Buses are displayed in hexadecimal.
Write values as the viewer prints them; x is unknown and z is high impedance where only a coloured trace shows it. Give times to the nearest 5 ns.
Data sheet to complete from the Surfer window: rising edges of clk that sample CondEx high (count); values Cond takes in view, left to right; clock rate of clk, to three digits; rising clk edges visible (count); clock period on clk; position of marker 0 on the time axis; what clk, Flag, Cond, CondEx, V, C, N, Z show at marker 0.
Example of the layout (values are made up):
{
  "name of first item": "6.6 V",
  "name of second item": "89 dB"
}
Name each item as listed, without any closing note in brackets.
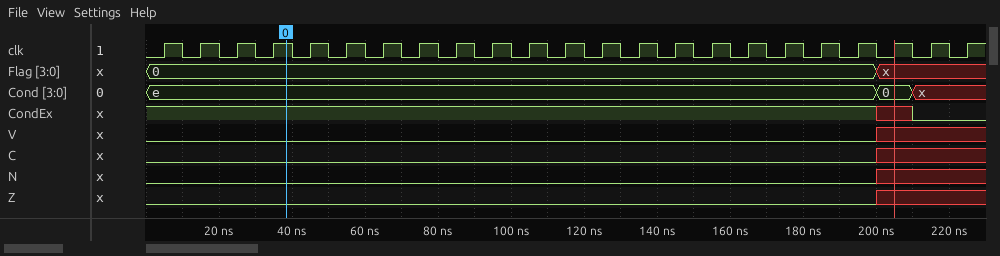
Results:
{
  "rising edges of clk that sample CondEx high": "20",
  "values Cond takes in view, left to right": "e, 0, x",
  "clock rate of clk, to three digits": "100 MHz",
  "rising clk edges visible": "23",
  "clock period on clk": "10 ns",
  "position of marker 0 on the time axis": "40 ns",
  "what clk, Flag, Cond, CondEx, V, C, N, Z show at marker 0": "clk=1, Flag=0, Cond=e, CondEx=1, V=0, C=0, N=0, Z=0"
}
